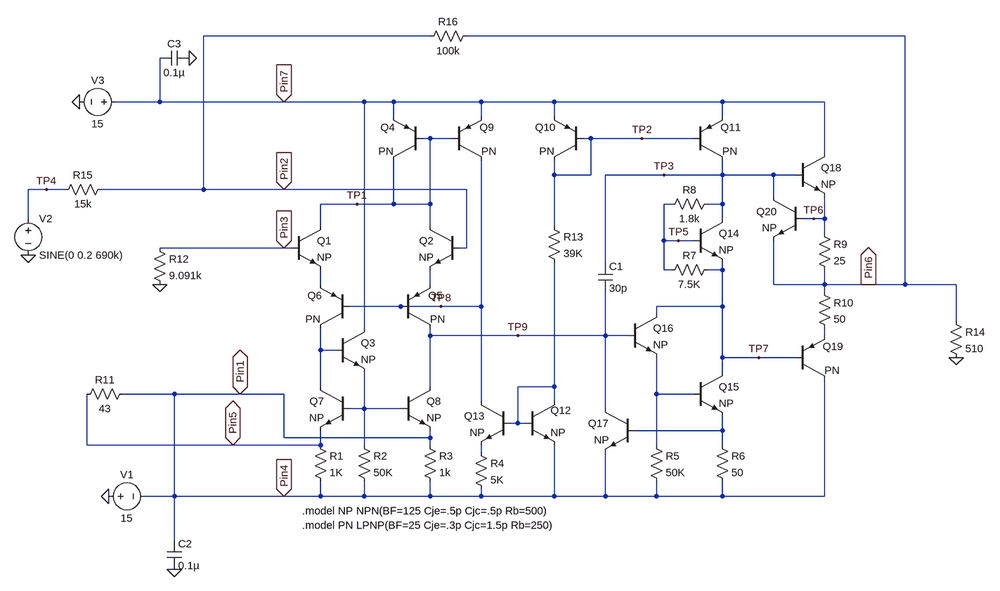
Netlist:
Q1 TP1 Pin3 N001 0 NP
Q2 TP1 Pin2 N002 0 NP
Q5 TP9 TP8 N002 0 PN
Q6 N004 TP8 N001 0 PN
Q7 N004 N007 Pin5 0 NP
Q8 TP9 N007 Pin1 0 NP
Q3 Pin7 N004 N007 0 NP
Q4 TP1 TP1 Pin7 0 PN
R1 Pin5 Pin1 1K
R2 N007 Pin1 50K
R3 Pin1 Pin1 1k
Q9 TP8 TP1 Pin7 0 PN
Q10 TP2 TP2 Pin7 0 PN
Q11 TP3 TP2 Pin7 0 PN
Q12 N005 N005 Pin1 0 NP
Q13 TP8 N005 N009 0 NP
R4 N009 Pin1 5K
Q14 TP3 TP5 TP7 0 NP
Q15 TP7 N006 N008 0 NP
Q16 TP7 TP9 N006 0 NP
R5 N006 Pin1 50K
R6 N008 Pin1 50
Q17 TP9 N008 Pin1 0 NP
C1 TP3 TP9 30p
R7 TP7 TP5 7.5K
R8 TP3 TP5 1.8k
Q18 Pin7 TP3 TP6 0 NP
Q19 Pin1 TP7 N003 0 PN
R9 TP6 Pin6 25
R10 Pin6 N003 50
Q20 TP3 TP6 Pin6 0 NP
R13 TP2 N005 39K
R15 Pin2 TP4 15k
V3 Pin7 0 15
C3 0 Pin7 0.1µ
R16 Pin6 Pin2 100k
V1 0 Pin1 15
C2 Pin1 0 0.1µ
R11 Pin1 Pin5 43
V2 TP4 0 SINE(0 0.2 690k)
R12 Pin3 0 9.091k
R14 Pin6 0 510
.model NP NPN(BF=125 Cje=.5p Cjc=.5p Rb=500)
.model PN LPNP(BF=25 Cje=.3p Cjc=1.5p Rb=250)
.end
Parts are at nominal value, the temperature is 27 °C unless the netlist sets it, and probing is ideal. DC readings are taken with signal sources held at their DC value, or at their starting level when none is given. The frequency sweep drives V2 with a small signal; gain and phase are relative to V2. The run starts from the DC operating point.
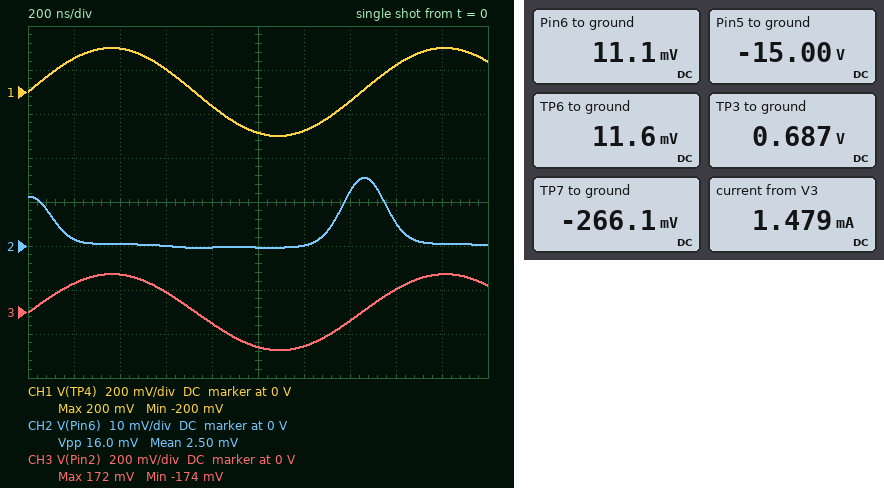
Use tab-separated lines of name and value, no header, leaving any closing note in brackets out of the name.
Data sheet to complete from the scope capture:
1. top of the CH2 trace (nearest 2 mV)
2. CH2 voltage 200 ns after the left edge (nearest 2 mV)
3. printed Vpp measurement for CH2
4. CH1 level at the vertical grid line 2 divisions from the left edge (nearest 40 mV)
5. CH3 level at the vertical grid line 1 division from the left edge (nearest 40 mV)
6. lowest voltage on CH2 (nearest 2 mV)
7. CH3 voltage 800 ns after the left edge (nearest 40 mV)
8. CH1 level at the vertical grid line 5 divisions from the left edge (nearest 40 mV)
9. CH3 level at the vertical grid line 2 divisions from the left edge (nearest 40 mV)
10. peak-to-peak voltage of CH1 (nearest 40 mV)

top of the CH2 trace	16 mV
CH2 voltage 200 ns after the left edge	2 mV
printed Vpp measurement for CH2	16.0 mV
CH1 level at the vertical grid line 2 divisions from the left edge	200 mV
CH3 level at the vertical grid line 1 division from the left edge	120 mV
lowest voltage on CH2	0 V
CH3 voltage 800 ns after the left edge	-40 mV
CH1 level at the vertical grid line 5 divisions from the left edge	-200 mV
CH3 level at the vertical grid line 2 divisions from the left edge	160 mV
peak-to-peak voltage of CH1	400 mV
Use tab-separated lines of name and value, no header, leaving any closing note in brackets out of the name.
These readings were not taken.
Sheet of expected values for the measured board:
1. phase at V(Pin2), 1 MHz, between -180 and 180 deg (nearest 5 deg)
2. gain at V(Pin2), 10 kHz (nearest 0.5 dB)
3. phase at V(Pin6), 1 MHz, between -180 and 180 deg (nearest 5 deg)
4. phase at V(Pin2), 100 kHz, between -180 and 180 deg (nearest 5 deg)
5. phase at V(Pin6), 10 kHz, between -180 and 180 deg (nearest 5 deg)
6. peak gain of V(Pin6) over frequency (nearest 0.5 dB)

phase at V(Pin2), 1 MHz, between -180 and 180 deg	0 deg
gain at V(Pin2), 10 kHz	-13.0 dB
phase at V(Pin6), 1 MHz, between -180 and 180 deg	85 deg
phase at V(Pin2), 100 kHz, between -180 and 180 deg	20 deg
phase at V(Pin6), 10 kHz, between -180 and 180 deg	165 deg
peak gain of V(Pin6) over frequency	16.5 dB
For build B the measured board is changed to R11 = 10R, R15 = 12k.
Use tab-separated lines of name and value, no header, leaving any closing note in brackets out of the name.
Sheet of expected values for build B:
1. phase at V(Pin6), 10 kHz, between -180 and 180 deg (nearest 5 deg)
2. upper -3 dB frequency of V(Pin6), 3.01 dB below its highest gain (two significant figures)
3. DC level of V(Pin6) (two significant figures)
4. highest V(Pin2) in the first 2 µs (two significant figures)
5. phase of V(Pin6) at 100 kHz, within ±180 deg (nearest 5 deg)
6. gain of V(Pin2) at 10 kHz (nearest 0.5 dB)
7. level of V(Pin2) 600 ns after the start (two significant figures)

phase at V(Pin6), 10 kHz, between -180 and 180 deg	155 deg
upper -3 dB frequency of V(Pin6), 3.01 dB below its highest gain	20 kHz
DC level of V(Pin6)	6.2 mV
highest V(Pin2) in the first 2 µs	180 mV
phase of V(Pin6) at 100 kHz, within ±180 deg	100 deg
gain of V(Pin2) at 10 kHz	-8.0 dB
level of V(Pin2) 600 ns after the start	92 mV
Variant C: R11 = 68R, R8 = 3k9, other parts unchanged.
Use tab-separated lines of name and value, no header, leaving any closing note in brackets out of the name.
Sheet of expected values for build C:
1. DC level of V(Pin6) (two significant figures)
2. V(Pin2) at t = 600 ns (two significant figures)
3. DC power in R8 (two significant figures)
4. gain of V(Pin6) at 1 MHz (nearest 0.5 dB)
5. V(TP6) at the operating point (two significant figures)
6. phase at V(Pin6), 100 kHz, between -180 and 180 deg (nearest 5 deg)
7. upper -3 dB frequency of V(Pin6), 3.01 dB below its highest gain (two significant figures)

DC level of V(Pin6)	14 mV
V(Pin2) at t = 600 ns	84 mV
DC power in R8	44 µW
gain of V(Pin6) at 1 MHz	-10.5 dB
V(TP6) at the operating point	15 mV
phase at V(Pin6), 100 kHz, between -180 and 180 deg	115 deg
upper -3 dB frequency of V(Pin6), 3.01 dB below its highest gain	45 kHz
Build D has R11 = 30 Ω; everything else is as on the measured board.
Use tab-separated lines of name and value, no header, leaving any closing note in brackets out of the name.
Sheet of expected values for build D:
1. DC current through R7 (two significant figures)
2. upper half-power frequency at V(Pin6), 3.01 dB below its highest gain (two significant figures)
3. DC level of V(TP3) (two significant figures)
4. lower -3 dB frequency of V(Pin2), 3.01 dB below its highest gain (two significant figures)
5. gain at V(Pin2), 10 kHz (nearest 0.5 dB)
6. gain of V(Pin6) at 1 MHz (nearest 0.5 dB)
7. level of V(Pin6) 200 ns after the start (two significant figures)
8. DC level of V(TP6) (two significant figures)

DC current through R7	100 µA
upper half-power frequency at V(Pin6), 3.01 dB below its highest gain	33 kHz
DC level of V(TP3)	680 mV
lower -3 dB frequency of V(Pin2), 3.01 dB below its highest gain	34 kHz
gain at V(Pin2), 10 kHz	-12.0 dB
gain of V(Pin6) at 1 MHz	-13.0 dB
level of V(Pin6) 200 ns after the start	1.2 mV
DC level of V(TP6)	9.8 mV
